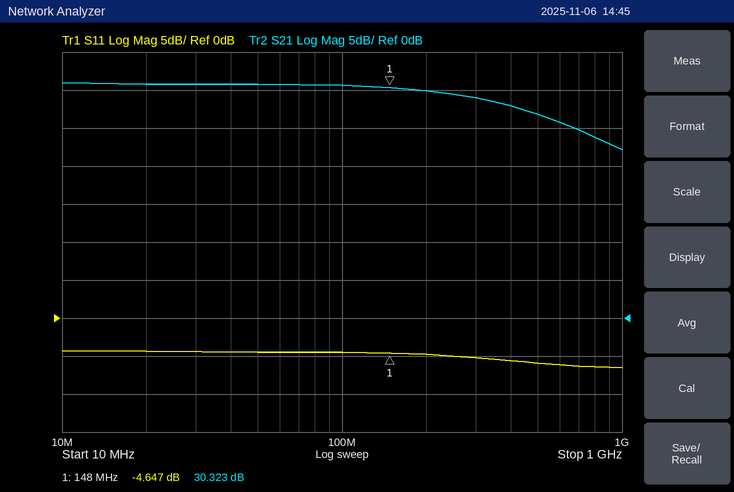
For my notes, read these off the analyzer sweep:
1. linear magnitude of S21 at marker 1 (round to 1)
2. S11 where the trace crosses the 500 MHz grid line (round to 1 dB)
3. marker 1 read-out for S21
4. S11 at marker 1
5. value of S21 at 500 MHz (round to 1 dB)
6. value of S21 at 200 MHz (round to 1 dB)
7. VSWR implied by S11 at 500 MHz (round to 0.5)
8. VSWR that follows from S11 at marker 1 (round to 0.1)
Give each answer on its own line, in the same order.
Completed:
33
-6 dB
30.323 dB
-4.647 dB
27 dB
30 dB
3.0
3.8
